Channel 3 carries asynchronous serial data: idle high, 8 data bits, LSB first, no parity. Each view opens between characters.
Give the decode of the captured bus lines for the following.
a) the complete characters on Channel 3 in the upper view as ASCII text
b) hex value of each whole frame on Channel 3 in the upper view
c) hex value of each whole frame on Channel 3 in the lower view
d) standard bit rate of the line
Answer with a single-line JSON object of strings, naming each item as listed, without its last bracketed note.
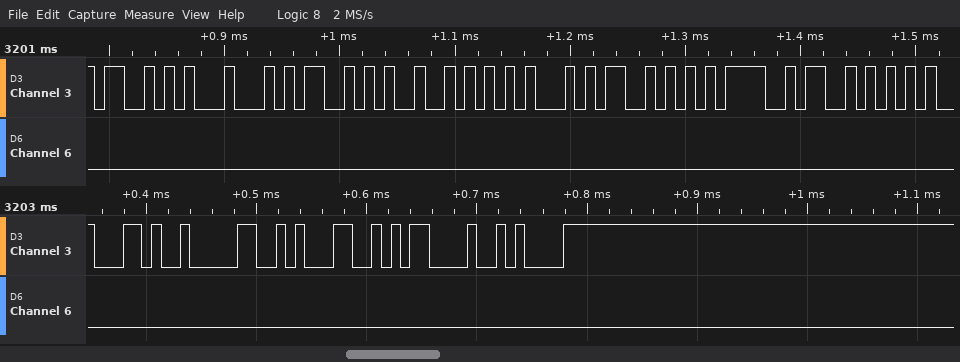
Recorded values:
{"the complete characters on Channel 3 in the upper view as ASCII text": "\"SDSRES=S\"", "hex value of each whole frame on Channel 3 in the upper view": "53, 44, 53, 52, 45, 53, 3D, 53", "hex value of each whole frame on Channel 3 in the lower view": "2C, 30, 31, 0D, 0A", "standard bit rate of the line": "115200 baud"}
